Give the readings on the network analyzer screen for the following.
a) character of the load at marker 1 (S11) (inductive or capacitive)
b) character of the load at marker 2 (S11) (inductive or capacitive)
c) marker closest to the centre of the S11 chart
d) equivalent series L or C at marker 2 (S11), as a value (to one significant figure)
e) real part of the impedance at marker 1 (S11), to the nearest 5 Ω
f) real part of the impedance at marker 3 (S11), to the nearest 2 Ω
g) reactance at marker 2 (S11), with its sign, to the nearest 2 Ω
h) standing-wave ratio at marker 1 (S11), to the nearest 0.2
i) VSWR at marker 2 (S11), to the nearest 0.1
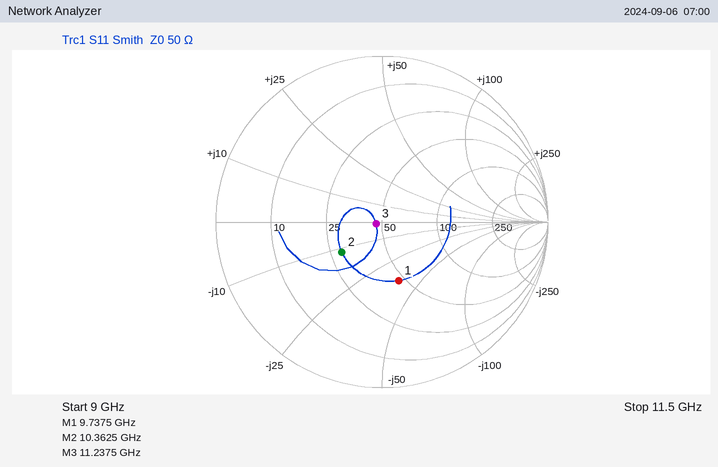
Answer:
capacitive
capacitive
marker 3
1 pF
45 Ω
46 Ω
-12 Ω
2.2
1.9
